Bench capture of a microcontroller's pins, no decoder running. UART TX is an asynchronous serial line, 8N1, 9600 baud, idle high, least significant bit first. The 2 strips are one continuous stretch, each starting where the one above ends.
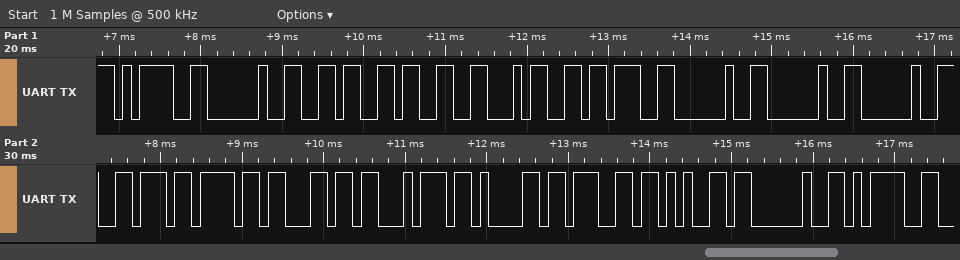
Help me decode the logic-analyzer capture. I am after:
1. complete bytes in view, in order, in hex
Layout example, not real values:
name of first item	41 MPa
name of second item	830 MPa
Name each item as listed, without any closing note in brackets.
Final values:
complete bytes in view, in order, in hex	3D 20 36 33 34 3B 20 20 20 76 6F 6C 74 61 67 65 20 3D
